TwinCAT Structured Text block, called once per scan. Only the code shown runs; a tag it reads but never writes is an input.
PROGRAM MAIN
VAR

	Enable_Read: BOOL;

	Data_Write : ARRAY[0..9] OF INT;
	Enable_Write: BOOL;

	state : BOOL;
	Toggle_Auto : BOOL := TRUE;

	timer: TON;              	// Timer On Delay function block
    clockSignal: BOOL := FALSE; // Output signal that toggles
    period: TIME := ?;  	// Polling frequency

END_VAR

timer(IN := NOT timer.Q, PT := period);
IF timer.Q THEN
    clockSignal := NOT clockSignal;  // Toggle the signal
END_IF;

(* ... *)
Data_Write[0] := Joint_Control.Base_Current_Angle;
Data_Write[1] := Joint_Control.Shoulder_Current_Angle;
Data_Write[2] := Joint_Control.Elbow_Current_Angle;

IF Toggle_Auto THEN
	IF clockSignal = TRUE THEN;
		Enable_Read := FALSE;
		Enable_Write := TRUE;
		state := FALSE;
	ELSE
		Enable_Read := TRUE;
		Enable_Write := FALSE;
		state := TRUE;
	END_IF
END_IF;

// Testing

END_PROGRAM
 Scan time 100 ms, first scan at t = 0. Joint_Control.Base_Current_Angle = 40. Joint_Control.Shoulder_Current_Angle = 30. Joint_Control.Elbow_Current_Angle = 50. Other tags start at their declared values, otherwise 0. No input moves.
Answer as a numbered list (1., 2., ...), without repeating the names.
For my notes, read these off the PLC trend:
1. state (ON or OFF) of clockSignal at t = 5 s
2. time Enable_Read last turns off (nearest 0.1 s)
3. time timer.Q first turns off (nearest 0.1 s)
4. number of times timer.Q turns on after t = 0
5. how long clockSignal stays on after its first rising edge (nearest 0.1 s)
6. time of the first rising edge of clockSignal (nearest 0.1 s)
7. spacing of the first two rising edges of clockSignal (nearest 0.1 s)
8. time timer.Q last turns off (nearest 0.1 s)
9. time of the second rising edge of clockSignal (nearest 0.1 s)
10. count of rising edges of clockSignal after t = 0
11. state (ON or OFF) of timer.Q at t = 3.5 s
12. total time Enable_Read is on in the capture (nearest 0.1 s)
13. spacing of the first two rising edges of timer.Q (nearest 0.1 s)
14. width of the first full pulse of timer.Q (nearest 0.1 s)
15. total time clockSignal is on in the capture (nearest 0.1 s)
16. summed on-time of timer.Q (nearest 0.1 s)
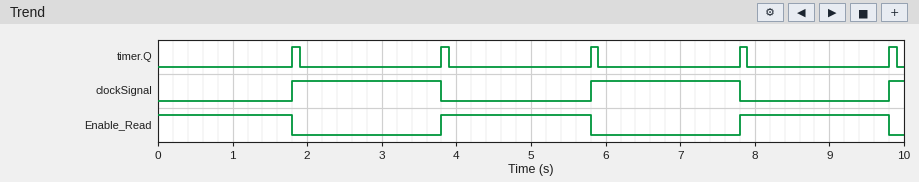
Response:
1. OFF
2. 9.8 s
3. 1.9 s
4. 5
5. 2.0 s
6. 1.8 s
7. 4.0 s
8. 9.9 s
9. 5.8 s
10. 3
11. OFF
12. 5.8 s
13. 2.0 s
14. 0.1 s
15. 4.2 s
16. 0.5 s
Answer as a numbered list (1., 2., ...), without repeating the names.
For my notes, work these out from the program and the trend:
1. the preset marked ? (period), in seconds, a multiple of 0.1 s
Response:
1. 1.8 s
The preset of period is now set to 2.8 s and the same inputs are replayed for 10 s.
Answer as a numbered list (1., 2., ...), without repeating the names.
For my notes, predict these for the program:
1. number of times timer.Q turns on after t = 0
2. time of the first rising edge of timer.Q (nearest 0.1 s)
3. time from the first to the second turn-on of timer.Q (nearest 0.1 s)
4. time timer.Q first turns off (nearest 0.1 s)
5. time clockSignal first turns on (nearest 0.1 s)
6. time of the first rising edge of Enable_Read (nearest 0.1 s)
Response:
1. 3
2. 2.8 s
3. 3.0 s
4. 2.9 s
5. 2.8 s
6. 5.8 s
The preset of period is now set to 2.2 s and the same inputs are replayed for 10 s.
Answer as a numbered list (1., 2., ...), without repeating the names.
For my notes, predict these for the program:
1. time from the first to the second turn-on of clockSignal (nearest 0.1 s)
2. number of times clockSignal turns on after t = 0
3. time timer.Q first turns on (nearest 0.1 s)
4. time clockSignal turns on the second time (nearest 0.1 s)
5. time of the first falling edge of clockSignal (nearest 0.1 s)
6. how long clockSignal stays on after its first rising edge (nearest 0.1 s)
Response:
1. 4.8 s
2. 2
3. 2.2 s
4. 7.0 s
5. 4.6 s
6. 2.4 s
